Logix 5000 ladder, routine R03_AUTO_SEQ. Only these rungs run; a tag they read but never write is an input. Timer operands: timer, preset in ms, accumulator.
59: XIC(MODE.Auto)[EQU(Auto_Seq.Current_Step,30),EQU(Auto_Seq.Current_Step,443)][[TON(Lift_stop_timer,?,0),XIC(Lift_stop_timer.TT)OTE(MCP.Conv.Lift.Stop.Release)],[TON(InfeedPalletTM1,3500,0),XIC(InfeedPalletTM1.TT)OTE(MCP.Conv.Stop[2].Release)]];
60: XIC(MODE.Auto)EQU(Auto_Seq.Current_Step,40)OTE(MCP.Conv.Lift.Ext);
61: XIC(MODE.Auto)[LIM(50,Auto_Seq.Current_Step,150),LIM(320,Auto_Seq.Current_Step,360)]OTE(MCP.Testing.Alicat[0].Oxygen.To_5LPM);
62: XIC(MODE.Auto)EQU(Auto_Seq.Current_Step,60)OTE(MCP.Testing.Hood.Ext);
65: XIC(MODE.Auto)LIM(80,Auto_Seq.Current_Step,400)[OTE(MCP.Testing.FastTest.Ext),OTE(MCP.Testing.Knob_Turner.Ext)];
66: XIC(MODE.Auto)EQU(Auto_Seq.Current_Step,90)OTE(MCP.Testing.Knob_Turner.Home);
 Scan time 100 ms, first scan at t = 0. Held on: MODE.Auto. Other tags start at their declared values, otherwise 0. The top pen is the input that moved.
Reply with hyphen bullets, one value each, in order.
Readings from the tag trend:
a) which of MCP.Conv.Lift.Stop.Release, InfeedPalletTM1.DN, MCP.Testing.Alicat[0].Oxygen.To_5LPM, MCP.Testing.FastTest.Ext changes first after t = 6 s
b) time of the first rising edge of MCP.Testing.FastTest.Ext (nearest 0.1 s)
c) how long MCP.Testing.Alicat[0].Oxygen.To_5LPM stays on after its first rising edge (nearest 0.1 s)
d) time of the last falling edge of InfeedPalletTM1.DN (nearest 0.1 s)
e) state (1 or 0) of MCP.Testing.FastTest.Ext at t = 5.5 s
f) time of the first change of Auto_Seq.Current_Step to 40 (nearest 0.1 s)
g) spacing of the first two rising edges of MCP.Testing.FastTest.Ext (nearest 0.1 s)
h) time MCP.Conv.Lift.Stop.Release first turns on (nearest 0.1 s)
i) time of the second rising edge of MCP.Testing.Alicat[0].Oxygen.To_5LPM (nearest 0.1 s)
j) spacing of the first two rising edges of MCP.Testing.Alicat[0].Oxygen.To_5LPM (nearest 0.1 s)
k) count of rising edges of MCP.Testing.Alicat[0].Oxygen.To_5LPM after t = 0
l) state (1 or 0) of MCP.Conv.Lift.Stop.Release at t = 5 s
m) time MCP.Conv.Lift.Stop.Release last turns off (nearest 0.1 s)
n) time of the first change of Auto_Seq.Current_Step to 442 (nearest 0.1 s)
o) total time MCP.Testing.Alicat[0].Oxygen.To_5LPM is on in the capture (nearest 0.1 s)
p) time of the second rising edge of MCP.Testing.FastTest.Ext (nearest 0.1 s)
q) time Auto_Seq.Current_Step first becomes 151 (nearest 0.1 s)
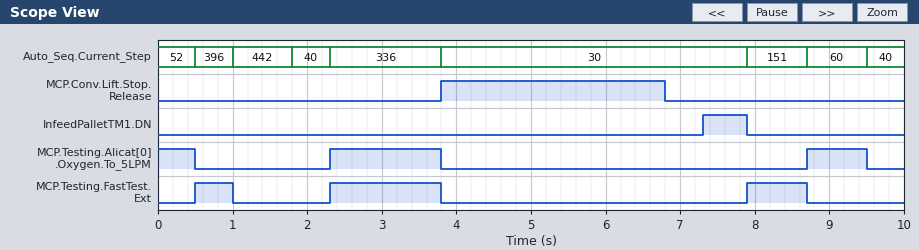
- MCP.Conv.Lift.Stop.Release
- 0.5 s
- 1.5 s
- 7.9 s
- 0
- 1.8 s
- 1.8 s
- 3.8 s
- 8.7 s
- 6.4 s
- 2
- 1
- 6.8 s
- 1.0 s
- 2.8 s
- 2.3 s
- 7.9 s
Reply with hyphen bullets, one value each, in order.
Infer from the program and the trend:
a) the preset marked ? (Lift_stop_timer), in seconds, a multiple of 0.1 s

- 3.0 s
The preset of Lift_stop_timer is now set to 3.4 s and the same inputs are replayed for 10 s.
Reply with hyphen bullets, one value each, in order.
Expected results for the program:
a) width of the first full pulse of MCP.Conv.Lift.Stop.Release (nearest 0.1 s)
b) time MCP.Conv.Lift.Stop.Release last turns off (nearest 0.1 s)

- 3.4 s
- 7.2 s
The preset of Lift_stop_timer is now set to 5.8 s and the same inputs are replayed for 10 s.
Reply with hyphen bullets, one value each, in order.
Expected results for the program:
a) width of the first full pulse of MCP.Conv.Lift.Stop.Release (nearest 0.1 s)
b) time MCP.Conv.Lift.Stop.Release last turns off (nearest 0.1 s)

- 4.1 s
- 7.9 s
